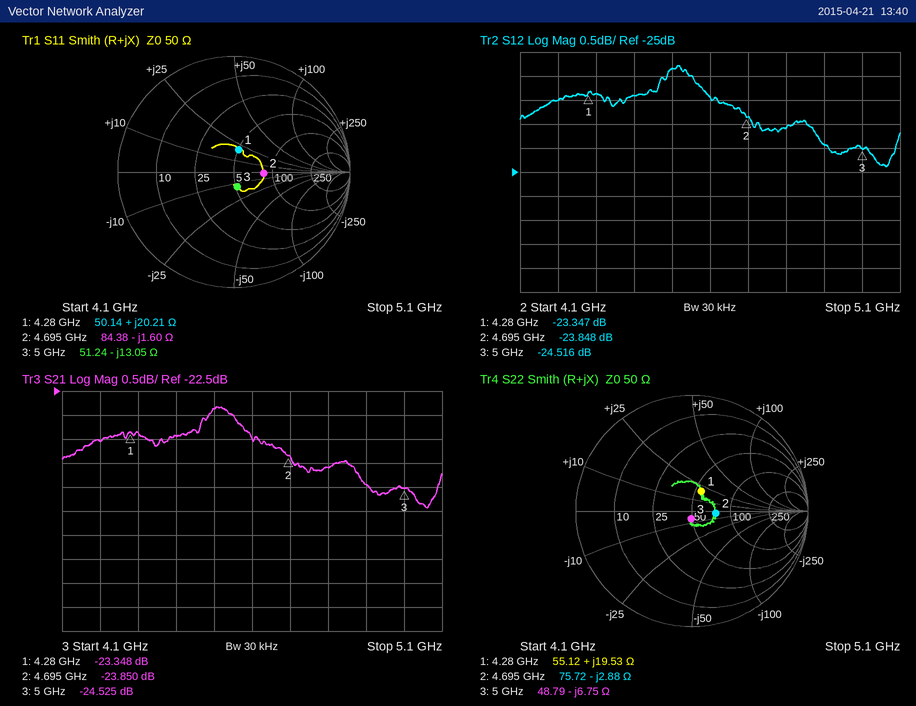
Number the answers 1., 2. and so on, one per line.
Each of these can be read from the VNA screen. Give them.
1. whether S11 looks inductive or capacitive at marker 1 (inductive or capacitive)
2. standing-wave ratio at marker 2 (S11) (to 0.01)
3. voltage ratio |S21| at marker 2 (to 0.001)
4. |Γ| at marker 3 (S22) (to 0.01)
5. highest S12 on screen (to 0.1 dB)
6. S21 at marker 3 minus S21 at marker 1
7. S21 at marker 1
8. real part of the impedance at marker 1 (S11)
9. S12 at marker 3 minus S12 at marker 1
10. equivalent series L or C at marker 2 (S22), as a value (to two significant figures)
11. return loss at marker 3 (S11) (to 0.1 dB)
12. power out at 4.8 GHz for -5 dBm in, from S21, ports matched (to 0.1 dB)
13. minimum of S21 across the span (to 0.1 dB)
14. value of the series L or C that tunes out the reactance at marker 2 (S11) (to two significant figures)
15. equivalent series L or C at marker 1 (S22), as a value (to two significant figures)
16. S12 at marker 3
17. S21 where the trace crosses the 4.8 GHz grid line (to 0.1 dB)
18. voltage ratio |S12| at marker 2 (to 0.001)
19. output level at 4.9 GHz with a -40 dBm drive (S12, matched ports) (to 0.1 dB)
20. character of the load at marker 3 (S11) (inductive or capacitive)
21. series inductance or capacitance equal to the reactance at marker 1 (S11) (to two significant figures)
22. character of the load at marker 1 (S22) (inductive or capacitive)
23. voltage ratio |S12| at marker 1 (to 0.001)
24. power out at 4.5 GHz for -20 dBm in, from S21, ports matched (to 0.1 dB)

1. inductive
2. 1.69
3. 0.064
4. 0.07
5. -22.8 dB
6. -1.177 dB
7. -23.348 dB
8. 50.14 Ω
9. -1.169 dB
10. 12 pF
11. 17.8 dB
12. -29.1 dBm
13. -24.9 dB
14. 54 pH
15. 730 pH
16. -24.516 dB
17. -24.1 dB
18. 0.064
19. -64.4 dBm
20. capacitive
21. 750 pH
22. inductive
23. 0.068
24. -42.9 dBm
